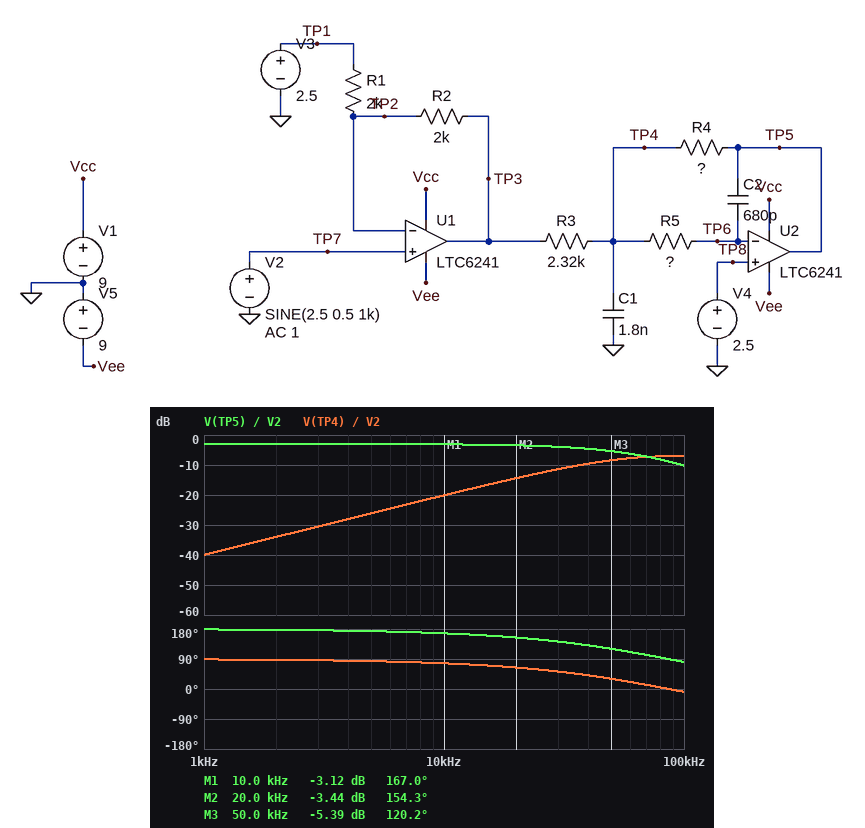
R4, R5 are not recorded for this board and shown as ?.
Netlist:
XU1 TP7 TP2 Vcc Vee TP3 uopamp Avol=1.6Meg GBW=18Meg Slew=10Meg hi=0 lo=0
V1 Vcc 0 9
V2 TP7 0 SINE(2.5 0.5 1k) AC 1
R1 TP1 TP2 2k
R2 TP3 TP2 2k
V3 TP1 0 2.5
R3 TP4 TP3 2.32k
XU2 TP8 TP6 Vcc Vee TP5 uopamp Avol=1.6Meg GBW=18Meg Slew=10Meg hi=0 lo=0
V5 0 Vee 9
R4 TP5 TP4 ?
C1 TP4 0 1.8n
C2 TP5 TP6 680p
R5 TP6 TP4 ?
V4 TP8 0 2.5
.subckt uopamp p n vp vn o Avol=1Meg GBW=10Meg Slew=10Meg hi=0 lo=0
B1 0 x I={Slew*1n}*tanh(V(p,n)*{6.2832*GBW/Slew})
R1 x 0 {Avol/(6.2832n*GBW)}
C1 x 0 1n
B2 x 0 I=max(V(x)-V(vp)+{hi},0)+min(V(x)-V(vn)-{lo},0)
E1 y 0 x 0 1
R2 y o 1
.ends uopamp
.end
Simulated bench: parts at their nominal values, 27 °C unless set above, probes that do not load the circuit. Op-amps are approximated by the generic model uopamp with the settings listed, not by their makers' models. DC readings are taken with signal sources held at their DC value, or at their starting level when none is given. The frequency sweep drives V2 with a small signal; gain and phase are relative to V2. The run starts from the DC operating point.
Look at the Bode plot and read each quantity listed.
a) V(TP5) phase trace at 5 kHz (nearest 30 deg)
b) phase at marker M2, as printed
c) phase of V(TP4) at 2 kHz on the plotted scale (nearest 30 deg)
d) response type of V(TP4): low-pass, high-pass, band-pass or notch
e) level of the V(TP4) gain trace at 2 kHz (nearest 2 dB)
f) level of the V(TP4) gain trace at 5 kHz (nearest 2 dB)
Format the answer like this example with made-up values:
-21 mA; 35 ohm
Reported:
180 deg; 154.3 deg; 90 deg; high-pass; -34 dB; -26 dB
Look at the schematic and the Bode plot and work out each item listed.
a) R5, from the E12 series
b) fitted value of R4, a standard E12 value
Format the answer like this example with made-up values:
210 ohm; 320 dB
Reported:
3.3 kΩ; 820 Ω
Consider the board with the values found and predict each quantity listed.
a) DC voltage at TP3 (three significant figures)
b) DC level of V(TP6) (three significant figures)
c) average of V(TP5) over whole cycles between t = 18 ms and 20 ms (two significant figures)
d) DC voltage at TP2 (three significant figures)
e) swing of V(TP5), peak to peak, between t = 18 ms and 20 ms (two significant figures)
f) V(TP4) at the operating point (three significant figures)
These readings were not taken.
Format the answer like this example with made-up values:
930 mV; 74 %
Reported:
2.50 V; 2.50 V; 2.5 V; 2.50 V; 710 mV; 2.50 V
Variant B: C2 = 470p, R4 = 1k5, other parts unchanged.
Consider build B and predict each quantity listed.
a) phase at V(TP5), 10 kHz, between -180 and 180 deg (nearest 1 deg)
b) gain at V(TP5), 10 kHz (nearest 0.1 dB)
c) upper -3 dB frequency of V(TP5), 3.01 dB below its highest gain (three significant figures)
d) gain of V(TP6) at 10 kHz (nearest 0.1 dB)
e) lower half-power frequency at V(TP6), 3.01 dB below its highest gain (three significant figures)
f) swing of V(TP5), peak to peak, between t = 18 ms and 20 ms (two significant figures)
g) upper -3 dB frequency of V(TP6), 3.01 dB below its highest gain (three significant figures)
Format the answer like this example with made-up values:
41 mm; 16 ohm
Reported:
168 deg; 2.2 dB; 68.0 kHz; -62.9 dB; 37.4 kHz; 1.3 V; 161 kHz
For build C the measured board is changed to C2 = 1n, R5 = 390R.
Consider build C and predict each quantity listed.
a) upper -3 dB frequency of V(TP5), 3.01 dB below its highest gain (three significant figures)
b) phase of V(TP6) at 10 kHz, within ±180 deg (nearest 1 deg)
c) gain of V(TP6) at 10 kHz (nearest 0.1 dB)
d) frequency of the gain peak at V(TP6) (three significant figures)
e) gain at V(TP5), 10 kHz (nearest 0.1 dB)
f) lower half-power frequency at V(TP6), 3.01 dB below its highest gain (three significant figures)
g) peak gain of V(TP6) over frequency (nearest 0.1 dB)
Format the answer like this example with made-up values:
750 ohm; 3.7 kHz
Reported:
159 kHz; 85 deg; -68.1 dB; 207 kHz; -3.0 dB; 93.7 kHz; -46.7 dB
